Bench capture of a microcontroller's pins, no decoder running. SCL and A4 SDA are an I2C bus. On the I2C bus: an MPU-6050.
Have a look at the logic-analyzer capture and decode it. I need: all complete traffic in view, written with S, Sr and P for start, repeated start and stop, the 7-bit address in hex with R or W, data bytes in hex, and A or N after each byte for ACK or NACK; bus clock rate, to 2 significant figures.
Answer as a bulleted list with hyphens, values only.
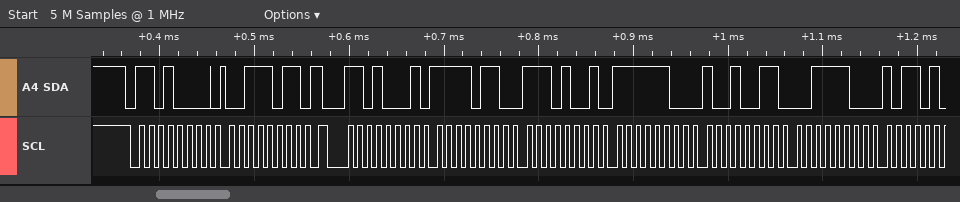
- S 68W A 3B A Sr 68R A F6 A E9 A FC A 93 A 3C A
- 100 kHz
